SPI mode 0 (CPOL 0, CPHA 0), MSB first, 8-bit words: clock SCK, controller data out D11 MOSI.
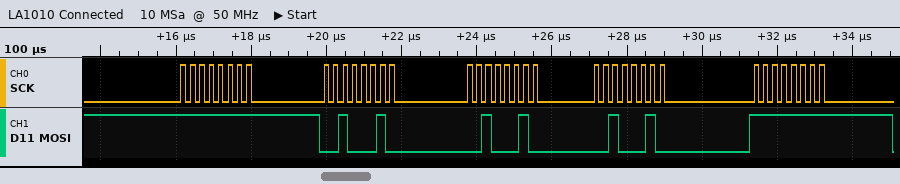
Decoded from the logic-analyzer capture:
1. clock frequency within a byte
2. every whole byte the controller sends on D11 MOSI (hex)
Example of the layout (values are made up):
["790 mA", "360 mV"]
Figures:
["4 MHz", "FF 22 22 22 FF"]
